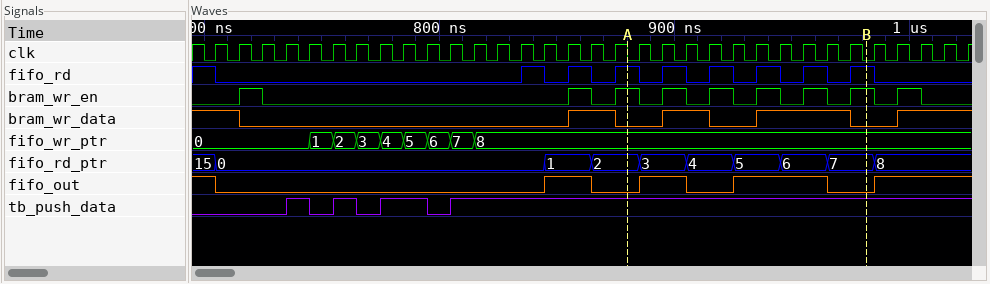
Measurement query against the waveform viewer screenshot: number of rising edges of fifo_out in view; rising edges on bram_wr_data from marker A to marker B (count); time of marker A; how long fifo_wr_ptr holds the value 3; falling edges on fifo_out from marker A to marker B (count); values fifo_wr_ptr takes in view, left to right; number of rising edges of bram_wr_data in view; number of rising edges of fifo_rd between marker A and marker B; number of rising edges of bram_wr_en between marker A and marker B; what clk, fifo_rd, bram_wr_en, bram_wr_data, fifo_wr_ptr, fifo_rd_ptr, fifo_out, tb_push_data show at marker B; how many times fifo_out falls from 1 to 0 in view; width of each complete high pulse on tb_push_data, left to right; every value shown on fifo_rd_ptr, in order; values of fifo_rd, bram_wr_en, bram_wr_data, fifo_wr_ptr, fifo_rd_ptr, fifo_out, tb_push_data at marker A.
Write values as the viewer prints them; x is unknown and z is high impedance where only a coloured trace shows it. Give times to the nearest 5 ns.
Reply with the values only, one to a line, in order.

4
2
880 ns
10 ns
2
0, 1, 2, 3, 4, 5, 6, 7, 8
4
5
5
clk=0, fifo_rd=1, bram_wr_en=1, bram_wr_data=0, fifo_wr_ptr=8, fifo_rd_ptr=7, fifo_out=0, tb_push_data=1
4
10 ns, 10 ns, 20 ns
15, 0, 1, 2, 3, 4, 5, 6, 7, 8
fifo_rd=1, bram_wr_en=1, bram_wr_data=0, fifo_wr_ptr=8, fifo_rd_ptr=2, fifo_out=0, tb_push_data=1
